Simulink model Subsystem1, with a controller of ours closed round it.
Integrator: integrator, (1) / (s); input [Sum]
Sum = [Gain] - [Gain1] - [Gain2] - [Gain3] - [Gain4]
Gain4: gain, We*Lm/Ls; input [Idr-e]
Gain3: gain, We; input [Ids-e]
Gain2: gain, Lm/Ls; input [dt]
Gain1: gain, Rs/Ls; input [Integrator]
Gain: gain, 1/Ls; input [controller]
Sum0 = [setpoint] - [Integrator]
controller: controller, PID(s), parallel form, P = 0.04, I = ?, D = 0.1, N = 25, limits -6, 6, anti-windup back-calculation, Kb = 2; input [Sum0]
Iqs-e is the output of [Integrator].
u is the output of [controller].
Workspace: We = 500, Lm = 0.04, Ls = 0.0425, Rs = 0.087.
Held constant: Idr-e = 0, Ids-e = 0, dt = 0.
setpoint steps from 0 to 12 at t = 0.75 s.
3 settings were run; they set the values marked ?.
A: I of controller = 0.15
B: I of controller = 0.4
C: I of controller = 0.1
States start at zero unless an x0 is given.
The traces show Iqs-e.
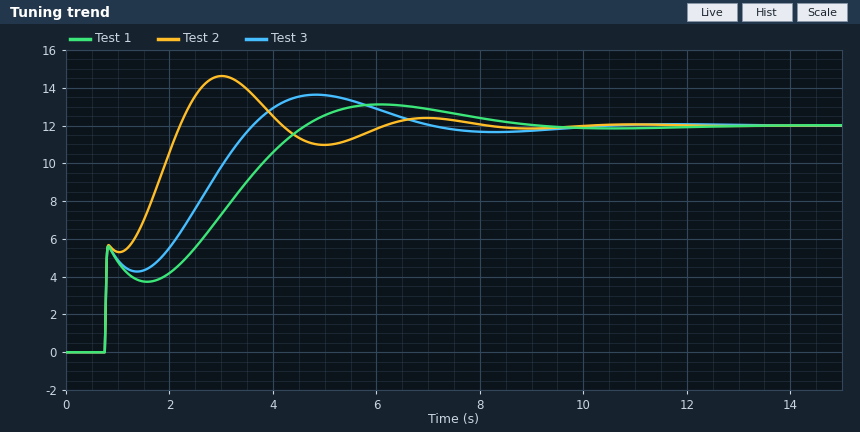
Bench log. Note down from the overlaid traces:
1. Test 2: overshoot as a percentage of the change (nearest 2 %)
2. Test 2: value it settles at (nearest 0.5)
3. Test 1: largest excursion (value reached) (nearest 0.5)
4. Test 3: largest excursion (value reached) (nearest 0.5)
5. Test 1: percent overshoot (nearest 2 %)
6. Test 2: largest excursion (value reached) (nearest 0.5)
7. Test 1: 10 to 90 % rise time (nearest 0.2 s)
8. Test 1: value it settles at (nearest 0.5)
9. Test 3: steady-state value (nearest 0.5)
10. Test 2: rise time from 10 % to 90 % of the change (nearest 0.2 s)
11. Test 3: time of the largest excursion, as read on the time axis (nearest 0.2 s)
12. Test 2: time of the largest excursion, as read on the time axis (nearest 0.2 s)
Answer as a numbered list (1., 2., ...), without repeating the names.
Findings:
1. 22 %
2. 12.0
3. 13.0
4. 13.5
5. 10 %
6. 14.5
7. 3.4 s
8. 12.0
9. 12.0
10. 1.2 s
11. 4.8 s
12. 3.0 s
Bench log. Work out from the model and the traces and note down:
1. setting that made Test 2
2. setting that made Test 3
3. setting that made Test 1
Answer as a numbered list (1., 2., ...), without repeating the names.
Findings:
1. B
2. A
3. C
